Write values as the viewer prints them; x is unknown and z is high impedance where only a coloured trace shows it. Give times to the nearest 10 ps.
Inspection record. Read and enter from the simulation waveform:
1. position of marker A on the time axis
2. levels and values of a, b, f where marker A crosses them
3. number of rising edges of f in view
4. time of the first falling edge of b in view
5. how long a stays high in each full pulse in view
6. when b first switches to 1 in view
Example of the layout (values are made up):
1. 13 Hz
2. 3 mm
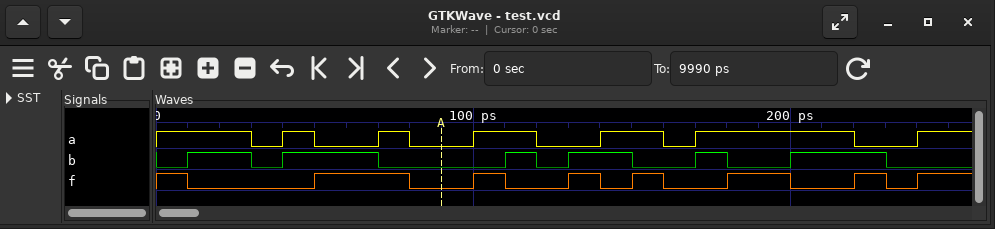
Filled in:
1. 90 ps
2. a=0, b=0, f=0
3. 7
4. 30 ps
5. 10 ps, 10 ps, 20 ps, 20 ps, 50 ps
6. 10 ps
